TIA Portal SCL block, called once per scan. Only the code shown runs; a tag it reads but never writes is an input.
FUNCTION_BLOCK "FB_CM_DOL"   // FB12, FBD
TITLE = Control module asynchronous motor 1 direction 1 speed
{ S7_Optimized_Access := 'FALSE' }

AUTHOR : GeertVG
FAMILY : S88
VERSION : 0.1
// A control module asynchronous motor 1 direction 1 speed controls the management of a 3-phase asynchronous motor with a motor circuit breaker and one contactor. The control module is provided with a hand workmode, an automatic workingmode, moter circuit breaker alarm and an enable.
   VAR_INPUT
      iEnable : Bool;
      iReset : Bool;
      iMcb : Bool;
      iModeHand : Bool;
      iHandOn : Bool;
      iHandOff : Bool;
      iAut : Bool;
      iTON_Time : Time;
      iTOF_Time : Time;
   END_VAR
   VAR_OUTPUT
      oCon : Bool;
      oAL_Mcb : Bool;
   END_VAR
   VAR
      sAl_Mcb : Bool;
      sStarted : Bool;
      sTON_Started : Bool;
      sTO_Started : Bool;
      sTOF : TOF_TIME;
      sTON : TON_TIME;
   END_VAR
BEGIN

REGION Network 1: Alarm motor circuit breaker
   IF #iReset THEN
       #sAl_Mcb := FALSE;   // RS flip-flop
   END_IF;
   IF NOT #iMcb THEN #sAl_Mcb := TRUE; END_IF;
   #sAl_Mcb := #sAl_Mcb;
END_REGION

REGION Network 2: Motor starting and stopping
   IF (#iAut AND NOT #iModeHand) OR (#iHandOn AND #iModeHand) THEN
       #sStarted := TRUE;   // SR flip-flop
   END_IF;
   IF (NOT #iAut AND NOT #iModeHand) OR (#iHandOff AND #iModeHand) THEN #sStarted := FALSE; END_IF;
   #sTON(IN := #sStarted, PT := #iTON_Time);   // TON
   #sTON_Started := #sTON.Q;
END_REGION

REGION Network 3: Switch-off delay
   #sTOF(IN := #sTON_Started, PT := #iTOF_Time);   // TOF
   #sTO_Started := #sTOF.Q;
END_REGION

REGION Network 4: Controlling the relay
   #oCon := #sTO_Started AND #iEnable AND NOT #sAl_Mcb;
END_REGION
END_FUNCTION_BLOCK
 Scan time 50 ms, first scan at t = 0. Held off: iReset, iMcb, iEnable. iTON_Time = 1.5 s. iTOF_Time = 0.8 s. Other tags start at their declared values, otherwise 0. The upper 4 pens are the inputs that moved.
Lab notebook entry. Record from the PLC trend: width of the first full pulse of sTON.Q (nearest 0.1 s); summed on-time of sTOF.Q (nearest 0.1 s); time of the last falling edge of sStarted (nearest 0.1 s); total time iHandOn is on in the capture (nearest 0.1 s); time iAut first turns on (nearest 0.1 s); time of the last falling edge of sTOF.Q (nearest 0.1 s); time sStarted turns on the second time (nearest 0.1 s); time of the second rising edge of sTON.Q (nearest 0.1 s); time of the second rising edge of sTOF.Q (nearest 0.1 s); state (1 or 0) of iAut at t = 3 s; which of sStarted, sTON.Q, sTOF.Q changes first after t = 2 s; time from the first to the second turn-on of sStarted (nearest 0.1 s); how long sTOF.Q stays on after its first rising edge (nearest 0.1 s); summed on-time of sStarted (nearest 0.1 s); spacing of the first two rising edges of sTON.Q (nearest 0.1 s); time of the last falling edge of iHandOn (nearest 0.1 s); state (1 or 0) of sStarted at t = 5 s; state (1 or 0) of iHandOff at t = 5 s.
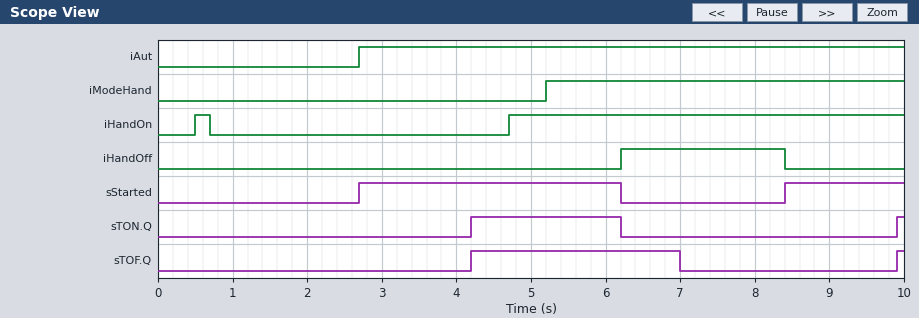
2.0 s
2.9 s
6.2 s
5.5 s
2.7 s
7.0 s
8.4 s
9.9 s
9.9 s
1
sStarted
5.7 s
2.8 s
5.1 s
5.7 s
0.7 s
1
0
